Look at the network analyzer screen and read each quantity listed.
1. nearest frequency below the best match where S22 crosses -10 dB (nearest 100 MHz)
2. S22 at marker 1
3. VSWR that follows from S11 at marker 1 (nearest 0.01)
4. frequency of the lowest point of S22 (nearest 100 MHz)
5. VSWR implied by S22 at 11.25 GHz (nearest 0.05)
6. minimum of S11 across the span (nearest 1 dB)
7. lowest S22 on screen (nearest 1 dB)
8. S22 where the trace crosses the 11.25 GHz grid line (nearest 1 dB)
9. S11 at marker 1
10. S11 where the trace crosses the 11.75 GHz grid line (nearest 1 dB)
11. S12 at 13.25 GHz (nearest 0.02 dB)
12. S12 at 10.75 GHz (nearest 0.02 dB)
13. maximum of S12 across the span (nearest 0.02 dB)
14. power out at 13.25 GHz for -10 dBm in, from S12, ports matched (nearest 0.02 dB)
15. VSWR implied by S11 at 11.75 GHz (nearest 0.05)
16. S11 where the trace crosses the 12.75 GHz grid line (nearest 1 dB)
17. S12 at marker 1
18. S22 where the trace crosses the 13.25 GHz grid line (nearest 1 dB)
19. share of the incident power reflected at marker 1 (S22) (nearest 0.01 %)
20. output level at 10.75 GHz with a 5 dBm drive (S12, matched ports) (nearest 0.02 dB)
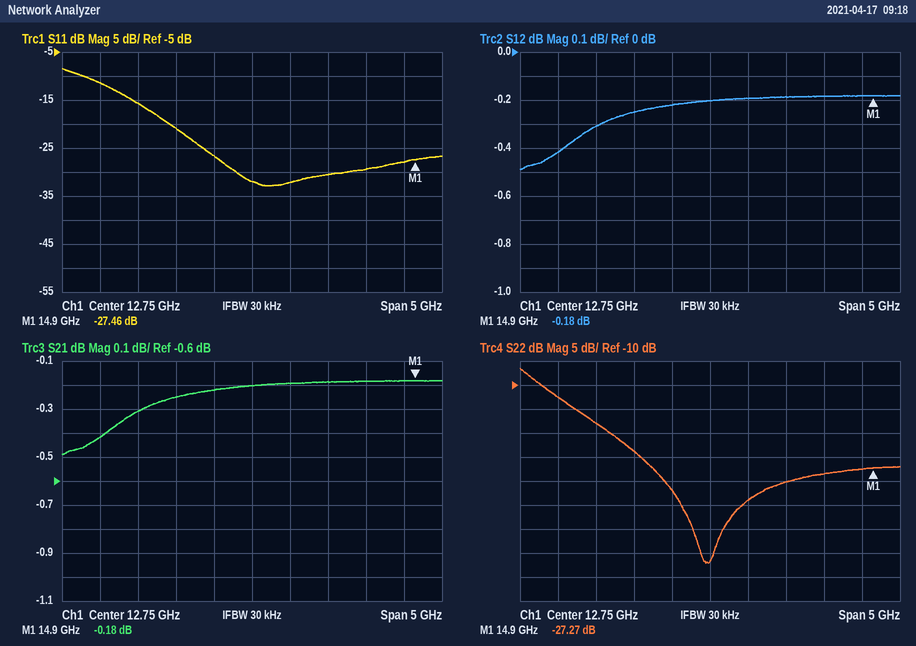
10.5 GHz
-27.27 dB
1.09
12.7 GHz
1.30
-33 dB
-47 dB
-18 dB
-27.46 dB
-21 dB
-0.20 dB
-0.42 dB
-0.18 dB
-10.20 dBm
1.20
-32 dB
-0.18 dB
-34 dB
0.19 %
4.58 dBm
